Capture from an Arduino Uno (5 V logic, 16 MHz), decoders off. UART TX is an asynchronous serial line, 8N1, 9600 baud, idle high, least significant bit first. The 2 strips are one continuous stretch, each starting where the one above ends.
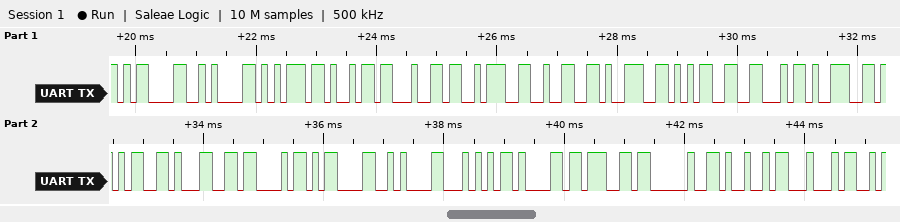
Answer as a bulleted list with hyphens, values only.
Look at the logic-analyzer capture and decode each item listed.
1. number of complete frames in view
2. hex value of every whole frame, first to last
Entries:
- 22
- 0x0D 0x0A 0x75 0x69 0x64 0x3A 0x32 0x39 0x35 0x46 0x39 0x35 0x31 0x43 0x0D 0x0A 0x54 0x61 0x67 0x20 0x49 0x44
